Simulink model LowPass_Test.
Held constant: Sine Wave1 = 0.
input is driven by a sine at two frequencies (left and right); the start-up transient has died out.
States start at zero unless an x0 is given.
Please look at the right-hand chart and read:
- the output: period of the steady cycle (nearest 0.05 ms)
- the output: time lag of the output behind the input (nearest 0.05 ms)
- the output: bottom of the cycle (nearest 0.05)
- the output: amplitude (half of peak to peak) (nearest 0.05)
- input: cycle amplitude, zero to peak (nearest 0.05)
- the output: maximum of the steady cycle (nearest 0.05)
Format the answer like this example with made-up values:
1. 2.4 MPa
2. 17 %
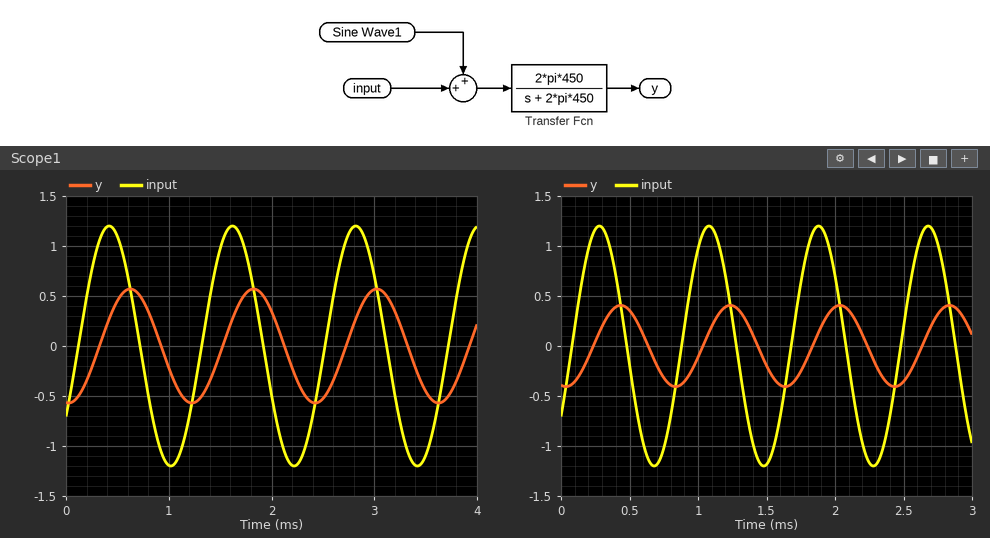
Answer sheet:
1. 0.80 ms
2. 0.15 ms
3. -0.40
4. 0.40
5. 1.20
6. 0.40
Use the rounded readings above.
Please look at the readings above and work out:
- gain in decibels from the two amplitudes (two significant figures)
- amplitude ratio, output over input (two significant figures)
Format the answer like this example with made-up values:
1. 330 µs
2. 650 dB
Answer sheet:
1. -9.5 dB
2. 0.33
